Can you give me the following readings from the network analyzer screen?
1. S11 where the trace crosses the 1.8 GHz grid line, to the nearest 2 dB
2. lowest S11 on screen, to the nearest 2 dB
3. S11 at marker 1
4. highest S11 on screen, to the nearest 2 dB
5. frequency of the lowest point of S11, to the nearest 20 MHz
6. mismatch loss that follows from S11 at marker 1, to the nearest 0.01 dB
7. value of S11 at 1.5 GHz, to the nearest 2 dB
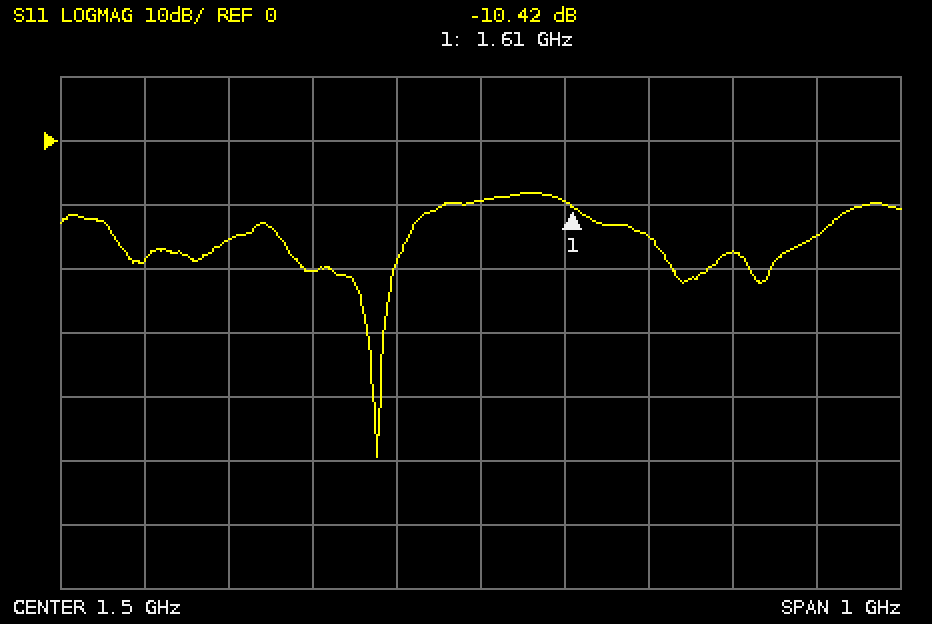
-18 dB
-50 dB
-10.42 dB
-8 dB
1.38 GHz
0.41 dB
-10 dB
